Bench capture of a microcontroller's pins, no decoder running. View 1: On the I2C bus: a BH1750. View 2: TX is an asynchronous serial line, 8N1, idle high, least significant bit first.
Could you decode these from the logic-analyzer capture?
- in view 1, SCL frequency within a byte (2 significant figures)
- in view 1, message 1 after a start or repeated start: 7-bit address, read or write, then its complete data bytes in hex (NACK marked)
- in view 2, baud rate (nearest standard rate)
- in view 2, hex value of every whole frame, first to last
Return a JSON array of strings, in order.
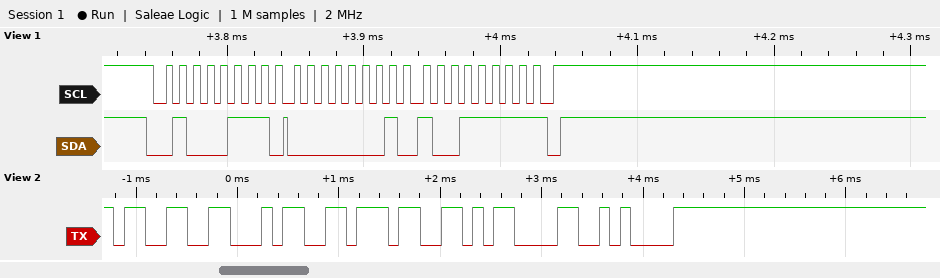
["100 kHz", "0x23 read: 01 9F NACK", "9600 baud", "33 34 37 0D 0A"]
